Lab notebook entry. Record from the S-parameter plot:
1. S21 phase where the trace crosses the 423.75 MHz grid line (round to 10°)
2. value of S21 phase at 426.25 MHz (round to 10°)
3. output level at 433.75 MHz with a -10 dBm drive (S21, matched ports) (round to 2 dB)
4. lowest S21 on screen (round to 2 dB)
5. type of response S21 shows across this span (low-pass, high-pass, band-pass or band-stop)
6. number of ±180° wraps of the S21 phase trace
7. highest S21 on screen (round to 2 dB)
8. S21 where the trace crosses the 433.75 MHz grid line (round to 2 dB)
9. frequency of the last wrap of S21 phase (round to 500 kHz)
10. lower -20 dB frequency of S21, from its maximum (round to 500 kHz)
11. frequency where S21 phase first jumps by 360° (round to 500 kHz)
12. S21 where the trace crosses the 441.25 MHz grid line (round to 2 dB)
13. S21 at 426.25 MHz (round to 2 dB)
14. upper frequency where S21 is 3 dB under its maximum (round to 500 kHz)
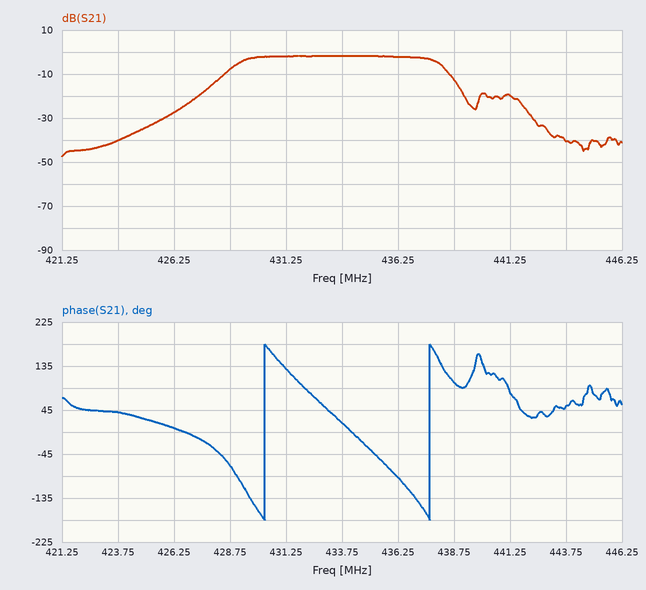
40°
10°
-12 dBm
-48 dB
band-pass
2
-2 dB
-2 dB
437.5 MHz
427.0 MHz
430.5 MHz
-20 dB
-28 dB
438.0 MHz
